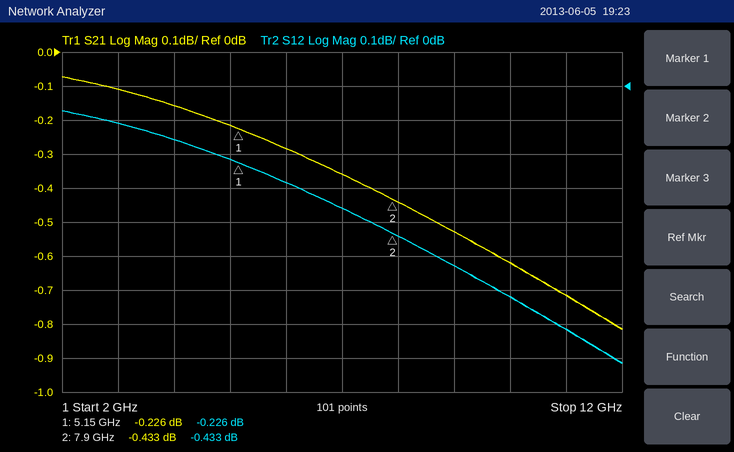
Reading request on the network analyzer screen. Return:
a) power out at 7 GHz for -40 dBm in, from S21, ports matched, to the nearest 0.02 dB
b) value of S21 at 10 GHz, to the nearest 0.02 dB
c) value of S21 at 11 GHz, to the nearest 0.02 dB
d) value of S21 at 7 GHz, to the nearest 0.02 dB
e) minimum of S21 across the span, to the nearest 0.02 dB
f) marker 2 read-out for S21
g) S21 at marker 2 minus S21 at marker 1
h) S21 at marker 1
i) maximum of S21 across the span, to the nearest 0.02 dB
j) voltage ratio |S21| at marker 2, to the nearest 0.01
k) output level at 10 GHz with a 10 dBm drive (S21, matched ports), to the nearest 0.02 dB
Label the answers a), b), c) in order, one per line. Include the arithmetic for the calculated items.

a) -40 dBm + (-0.36 dB) = -40.36 dBm
b) -0.62 dB
c) -0.72 dB
d) -0.36 dB
e) -0.82 dB
f) -0.433 dB
g) -0.433 − (-0.226) = -0.207 dB
h) -0.226 dB
i) -0.08 dB
j) 10^(-0.433/20) ≈ 0.95
k) 10 dBm + (-0.62 dB) = 9.38 dBm
